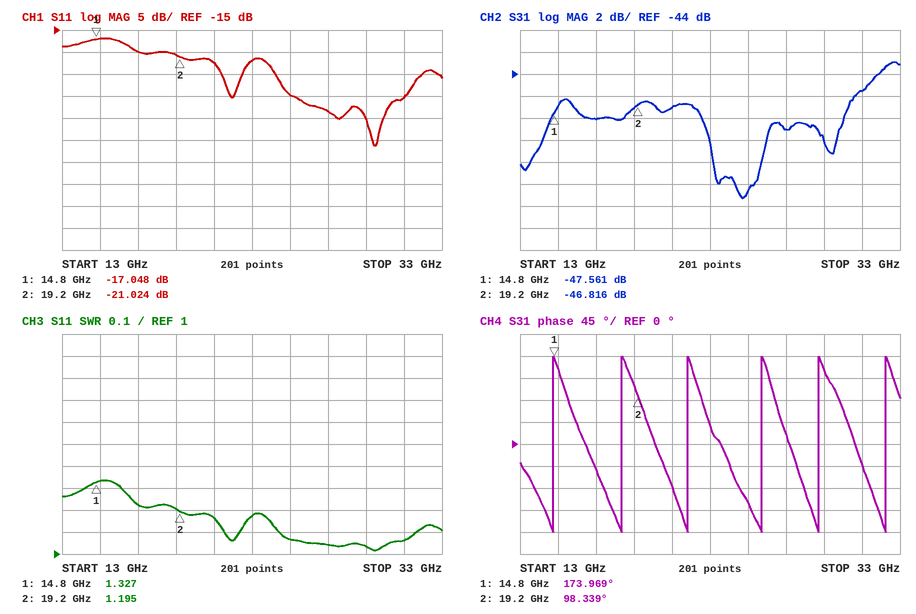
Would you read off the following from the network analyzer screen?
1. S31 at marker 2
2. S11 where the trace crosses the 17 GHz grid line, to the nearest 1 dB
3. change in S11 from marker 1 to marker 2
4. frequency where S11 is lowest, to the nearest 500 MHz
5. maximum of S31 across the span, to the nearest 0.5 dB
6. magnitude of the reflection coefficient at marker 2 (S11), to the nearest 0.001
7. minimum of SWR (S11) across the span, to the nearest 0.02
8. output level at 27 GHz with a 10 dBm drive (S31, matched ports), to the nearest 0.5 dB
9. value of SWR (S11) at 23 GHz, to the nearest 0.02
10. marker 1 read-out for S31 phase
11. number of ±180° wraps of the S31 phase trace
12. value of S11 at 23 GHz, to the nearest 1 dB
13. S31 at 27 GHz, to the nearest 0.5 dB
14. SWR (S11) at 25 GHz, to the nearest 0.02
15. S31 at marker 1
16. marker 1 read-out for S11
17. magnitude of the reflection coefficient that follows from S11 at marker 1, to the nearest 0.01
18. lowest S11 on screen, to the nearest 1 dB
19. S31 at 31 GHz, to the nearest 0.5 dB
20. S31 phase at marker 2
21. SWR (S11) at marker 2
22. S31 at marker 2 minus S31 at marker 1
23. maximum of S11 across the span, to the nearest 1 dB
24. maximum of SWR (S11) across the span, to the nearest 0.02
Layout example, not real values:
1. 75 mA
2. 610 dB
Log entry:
1. -46.816 dB
2. -20 dB
3. -3.976 dB
4. 29.5 GHz
5. -43.0 dB
6. 0.089
7. 1.02
8. -39.0 dBm
9. 1.18
10. 173.969°
11. 6
12. -22 dB
13. -49.0 dB
14. 1.06
15. -47.561 dB
16. -17.048 dB
17. 0.14
18. -41 dB
19. -45.5 dB
20. 98.339°
21. 1.195
22. 0.745 dB
23. -17 dB
24. 1.34
